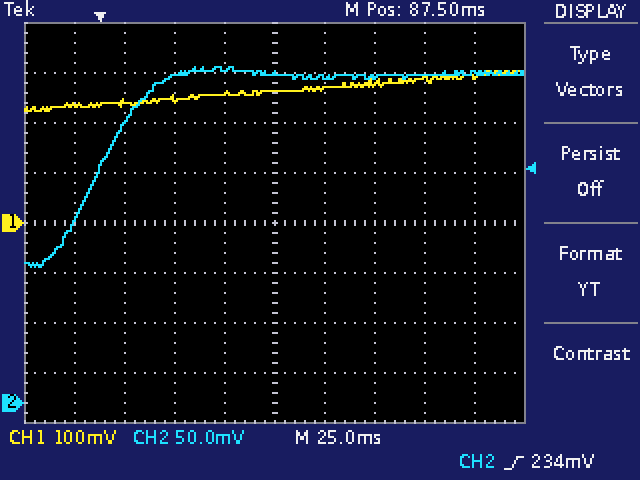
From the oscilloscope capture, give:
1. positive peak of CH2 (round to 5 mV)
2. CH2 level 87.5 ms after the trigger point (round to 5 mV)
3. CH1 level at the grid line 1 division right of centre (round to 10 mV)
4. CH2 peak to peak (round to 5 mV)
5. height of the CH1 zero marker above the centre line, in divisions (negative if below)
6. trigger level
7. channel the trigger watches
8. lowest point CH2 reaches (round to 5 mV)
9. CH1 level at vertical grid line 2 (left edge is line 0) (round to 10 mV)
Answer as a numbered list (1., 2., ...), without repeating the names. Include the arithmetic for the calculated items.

1. 335 mV
2. 330 mV
3. 270 mV
4. 335 mV − (135 mV) = 200 mV
5. 0.0 div
6. 234 mV
7. CH2
8. 135 mV
9. 240 mV
